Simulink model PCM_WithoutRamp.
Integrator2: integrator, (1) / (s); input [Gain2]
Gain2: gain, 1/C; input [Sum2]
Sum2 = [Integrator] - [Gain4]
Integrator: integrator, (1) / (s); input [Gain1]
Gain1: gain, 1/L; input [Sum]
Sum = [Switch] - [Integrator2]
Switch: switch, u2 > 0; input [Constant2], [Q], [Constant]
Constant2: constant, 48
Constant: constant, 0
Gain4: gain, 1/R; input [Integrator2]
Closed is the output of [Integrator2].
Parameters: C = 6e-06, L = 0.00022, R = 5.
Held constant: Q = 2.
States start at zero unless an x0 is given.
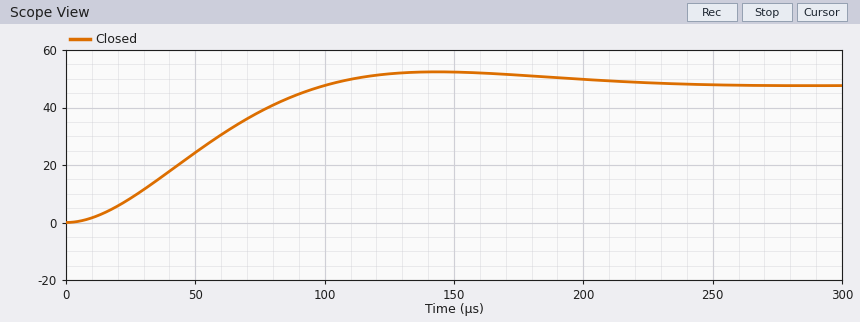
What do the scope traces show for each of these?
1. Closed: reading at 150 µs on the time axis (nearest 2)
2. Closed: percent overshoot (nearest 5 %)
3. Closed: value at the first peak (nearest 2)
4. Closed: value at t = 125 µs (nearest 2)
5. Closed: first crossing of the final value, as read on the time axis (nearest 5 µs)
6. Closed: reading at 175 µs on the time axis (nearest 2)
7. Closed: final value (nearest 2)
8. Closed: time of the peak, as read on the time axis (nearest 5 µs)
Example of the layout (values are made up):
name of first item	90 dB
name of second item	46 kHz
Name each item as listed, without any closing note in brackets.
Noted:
Closed: reading at 150 µs on the time axis	52
Closed: percent overshoot	10 %
Closed: value at the first peak	52
Closed: value at t = 125 µs	52
Closed: first crossing of the final value, as read on the time axis	100 µs
Closed: reading at 175 µs on the time axis	52
Closed: final value	48
Closed: time of the peak, as read on the time axis	145 µs
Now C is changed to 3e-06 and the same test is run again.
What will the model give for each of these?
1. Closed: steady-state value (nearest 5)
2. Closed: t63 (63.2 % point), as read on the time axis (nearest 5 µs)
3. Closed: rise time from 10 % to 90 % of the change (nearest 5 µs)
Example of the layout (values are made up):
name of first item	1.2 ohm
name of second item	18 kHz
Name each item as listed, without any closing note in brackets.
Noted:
Closed: steady-state value	50
Closed: t63 (63.2 % point), as read on the time axis	50 µs
Closed: rise time from 10 % to 90 % of the change	70 µs
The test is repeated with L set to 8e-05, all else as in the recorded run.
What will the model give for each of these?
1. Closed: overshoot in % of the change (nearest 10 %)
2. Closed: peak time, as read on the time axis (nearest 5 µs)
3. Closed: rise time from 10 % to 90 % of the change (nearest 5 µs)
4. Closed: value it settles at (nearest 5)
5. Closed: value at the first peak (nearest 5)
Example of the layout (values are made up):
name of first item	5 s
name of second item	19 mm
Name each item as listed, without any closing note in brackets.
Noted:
Closed: overshoot in % of the change	30 %
Closed: peak time, as read on the time axis	75 µs
Closed: rise time from 10 % to 90 % of the change	30 µs
Closed: value it settles at	50
Closed: value at the first peak	60
